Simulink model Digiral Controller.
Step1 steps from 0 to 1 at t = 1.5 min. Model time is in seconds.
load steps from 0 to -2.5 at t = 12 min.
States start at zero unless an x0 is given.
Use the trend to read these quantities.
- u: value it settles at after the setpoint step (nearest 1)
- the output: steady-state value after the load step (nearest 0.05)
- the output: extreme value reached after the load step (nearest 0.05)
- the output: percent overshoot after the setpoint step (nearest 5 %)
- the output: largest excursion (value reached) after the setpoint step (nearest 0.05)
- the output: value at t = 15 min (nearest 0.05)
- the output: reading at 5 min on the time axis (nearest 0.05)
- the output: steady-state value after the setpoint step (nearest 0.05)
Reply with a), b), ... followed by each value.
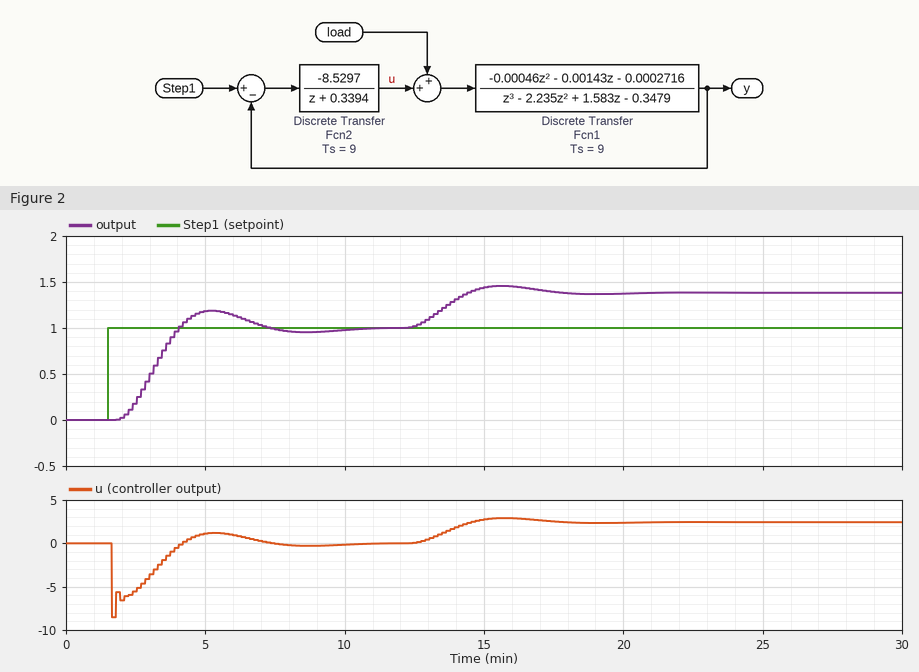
a) 0
b) 1.40
c) 1.45
d) 20 %
e) 1.20
f) 1.45
g) 1.20
h) 1.00
